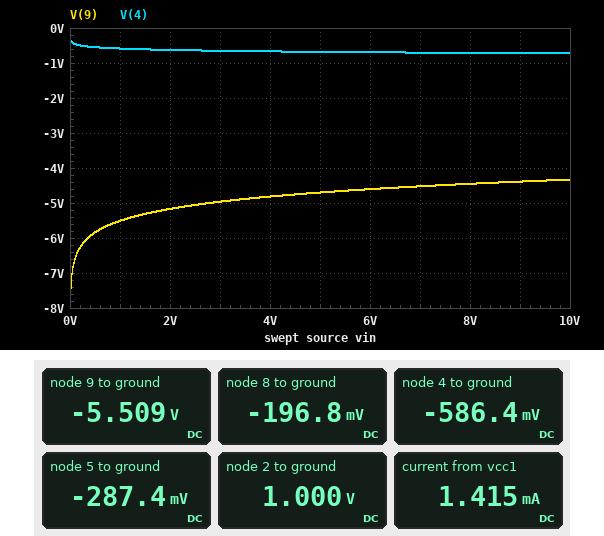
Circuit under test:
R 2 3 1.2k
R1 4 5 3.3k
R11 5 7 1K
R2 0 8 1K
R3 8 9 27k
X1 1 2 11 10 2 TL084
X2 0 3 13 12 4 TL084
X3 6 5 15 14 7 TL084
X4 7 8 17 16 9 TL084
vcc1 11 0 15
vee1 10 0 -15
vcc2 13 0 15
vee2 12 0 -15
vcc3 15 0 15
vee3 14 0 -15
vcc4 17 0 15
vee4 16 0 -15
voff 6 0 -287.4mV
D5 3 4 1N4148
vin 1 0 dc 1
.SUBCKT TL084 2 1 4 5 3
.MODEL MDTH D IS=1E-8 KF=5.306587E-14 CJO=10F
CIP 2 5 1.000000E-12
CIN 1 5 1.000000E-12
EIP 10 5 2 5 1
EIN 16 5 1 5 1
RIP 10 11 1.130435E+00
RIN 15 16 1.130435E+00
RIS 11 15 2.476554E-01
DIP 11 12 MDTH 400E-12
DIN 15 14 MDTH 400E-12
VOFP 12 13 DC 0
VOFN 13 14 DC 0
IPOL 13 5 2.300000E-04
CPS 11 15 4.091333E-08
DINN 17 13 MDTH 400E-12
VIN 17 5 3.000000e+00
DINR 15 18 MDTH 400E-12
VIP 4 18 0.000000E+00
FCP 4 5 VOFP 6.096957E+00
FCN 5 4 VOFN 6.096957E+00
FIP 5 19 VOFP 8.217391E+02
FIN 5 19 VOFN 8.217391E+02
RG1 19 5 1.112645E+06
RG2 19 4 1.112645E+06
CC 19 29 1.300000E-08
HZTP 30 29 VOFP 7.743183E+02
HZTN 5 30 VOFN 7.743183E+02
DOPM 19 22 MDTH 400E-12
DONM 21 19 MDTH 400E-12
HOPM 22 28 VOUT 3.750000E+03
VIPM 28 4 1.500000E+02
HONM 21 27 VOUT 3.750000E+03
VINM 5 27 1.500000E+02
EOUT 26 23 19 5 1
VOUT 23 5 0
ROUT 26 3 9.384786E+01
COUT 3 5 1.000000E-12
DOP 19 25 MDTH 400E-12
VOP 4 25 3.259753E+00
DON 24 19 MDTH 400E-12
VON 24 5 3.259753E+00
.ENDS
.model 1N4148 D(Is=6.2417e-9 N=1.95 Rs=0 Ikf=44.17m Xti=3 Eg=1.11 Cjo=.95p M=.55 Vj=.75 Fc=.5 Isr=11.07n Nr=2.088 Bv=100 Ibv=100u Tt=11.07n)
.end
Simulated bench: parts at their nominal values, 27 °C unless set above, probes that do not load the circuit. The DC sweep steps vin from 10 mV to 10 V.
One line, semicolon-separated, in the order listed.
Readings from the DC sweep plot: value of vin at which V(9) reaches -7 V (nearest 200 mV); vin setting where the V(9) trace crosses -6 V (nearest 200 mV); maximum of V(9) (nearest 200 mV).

0 V; 400 mV; -4.4 V
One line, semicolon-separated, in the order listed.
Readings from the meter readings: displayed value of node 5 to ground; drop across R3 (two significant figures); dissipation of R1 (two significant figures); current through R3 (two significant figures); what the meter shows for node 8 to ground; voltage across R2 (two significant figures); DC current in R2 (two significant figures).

-287.4 mV; 5.3 V; 27 µW; 200 µA; -196.8 mV; 200 mV; 200 µA
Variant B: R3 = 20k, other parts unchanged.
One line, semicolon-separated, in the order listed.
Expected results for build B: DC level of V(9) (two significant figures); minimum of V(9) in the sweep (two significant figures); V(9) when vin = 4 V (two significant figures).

-4.1 V; -5.7 V; -3.6 V
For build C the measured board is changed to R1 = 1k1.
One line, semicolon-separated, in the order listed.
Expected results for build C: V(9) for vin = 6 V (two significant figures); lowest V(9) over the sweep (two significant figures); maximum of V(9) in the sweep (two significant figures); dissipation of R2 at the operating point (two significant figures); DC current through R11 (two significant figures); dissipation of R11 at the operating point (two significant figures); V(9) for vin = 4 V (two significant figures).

2.3 V; -6.9 V; 3.1 V; 240 nW; 270 µA; 74 µW; 1.6 V
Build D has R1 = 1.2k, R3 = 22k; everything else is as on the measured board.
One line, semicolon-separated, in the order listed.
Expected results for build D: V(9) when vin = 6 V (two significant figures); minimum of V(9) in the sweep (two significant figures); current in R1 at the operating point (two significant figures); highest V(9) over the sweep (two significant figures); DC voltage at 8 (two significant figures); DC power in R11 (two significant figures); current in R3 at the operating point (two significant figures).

1.2 V; -5.7 V; 250 µA; 1.8 V; -38 mV; 62 µW; 38 µA
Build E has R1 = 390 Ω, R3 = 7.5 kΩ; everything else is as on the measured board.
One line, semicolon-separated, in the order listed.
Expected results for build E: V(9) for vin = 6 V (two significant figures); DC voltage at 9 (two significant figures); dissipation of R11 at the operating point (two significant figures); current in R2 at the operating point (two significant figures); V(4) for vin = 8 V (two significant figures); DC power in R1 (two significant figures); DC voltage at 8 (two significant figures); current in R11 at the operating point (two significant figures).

6.4 V; 4.1 V; 590 µW; 480 µA; -710 mV; 230 µW; 480 mV; 770 µA
